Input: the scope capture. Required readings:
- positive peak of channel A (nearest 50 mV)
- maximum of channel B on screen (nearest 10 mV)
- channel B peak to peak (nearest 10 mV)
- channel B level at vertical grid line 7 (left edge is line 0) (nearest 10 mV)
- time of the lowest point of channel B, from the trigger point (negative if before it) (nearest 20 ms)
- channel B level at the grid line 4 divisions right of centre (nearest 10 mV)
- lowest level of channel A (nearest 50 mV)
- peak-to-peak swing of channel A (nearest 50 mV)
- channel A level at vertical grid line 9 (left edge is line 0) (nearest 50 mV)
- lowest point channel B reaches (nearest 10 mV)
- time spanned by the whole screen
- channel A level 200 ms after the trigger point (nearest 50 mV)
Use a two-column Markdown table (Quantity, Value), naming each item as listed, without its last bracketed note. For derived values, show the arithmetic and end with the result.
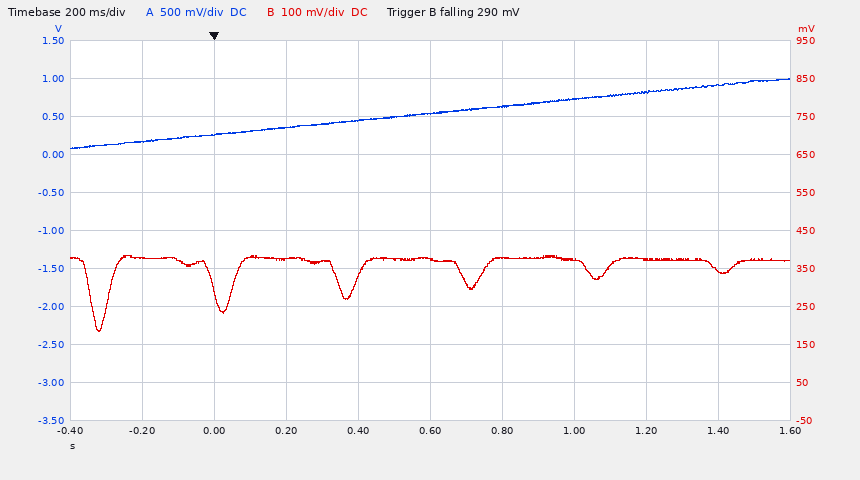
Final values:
| Quantity | Value |
|---|---|
| positive peak of channel A | 1.00 V |
| maximum of channel B on screen | 380 mV |
| channel B peak to peak | 380 mV − (180 mV) = 200 mV |
| channel B level at vertical grid line 7 (left edge is line 0) | 370 mV |
| time of the lowest point of channel B, from the trigger point (negative if before it) | -320 ms |
| channel B level at the grid line 4 divisions right of centre | 340 mV |
| lowest level of channel A | 100 mV |
| peak-to-peak swing of channel A | 1.00 V − (100 mV) = 900 mV |
| channel A level at vertical grid line 9 (left edge is line 0) | 900 mV |
| lowest point channel B reaches | 180 mV |
| time spanned by the whole screen | 2 s |
| channel A level 200 ms after the trigger point | 350 mV |
